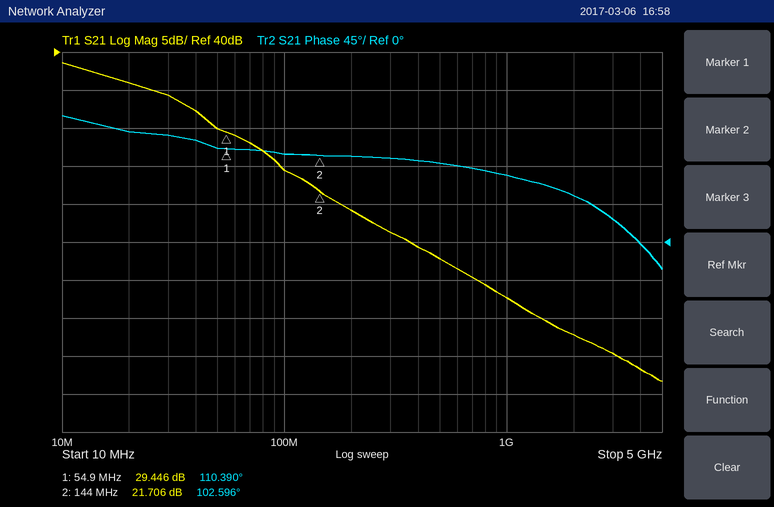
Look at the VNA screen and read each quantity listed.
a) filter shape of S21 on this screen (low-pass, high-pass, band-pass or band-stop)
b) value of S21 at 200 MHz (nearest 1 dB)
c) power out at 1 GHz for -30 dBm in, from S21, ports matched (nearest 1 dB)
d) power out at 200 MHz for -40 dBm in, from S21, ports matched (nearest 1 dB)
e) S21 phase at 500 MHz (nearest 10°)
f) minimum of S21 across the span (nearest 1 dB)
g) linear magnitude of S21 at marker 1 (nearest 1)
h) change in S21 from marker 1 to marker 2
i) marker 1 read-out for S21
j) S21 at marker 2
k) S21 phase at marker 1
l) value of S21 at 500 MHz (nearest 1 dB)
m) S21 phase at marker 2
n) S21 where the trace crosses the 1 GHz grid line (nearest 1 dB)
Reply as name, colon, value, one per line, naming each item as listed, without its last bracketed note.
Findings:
filter shape of S21 on this screen: low-pass
value of S21 at 200 MHz: 19 dB
power out at 1 GHz for -30 dBm in, from S21, ports matched: -22 dBm
power out at 200 MHz for -40 dBm in, from S21, ports matched: -21 dBm
S21 phase at 500 MHz: 90°
minimum of S21 across the span: -3 dB
linear magnitude of S21 at marker 1: 30
change in S21 from marker 1 to marker 2: -7.740 dB
marker 1 read-out for S21: 29.446 dB
S21 at marker 2: 21.706 dB
S21 phase at marker 1: 110.390°
value of S21 at 500 MHz: 13 dB
S21 phase at marker 2: 102.596°
S21 where the trace crosses the 1 GHz grid line: 8 dB
